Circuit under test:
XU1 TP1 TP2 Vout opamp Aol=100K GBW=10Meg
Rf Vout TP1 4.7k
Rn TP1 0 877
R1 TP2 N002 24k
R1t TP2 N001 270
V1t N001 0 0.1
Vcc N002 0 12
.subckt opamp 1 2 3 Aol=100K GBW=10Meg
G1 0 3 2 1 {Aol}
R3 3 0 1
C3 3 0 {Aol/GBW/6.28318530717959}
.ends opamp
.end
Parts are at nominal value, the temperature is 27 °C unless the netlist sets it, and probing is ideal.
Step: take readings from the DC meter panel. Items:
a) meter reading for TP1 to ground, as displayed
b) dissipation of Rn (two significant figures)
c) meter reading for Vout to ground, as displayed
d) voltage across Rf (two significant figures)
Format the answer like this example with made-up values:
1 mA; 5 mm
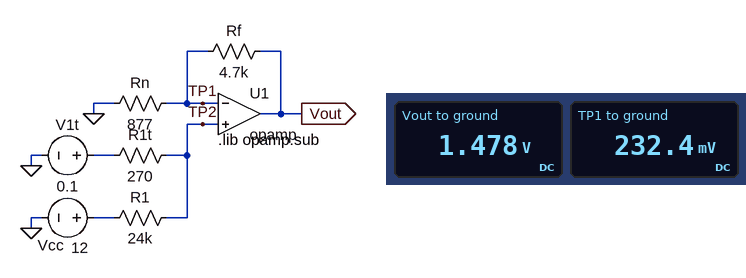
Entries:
232.4 mV; 62 µW; 1.478 V; 1.2 V
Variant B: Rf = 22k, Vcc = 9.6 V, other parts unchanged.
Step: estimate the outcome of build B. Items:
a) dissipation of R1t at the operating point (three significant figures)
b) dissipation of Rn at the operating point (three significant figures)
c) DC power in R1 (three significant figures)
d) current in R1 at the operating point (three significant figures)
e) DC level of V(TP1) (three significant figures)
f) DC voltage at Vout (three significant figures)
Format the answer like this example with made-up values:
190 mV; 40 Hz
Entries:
41.4 µW; 48.2 µW; 3.68 mW; 391 µA; 206 mV; 5.36 V
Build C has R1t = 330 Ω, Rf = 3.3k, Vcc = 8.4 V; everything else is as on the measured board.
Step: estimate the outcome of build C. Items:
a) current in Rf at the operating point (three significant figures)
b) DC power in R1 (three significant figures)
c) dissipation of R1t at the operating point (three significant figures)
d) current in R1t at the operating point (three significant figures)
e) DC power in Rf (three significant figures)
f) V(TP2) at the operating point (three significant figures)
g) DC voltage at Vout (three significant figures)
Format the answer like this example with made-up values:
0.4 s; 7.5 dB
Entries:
242 µA; 2.79 mW; 38.4 µW; 341 µA; 194 µW; 213 mV; 1.01 V
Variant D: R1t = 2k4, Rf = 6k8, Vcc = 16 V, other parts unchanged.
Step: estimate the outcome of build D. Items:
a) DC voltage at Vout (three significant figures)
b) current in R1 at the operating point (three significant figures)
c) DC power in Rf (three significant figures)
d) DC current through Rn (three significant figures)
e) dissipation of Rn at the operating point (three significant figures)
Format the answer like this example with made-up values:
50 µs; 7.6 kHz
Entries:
13.5 V; 602 µA; 21.1 mW; 1.76 mA; 2.72 mW
